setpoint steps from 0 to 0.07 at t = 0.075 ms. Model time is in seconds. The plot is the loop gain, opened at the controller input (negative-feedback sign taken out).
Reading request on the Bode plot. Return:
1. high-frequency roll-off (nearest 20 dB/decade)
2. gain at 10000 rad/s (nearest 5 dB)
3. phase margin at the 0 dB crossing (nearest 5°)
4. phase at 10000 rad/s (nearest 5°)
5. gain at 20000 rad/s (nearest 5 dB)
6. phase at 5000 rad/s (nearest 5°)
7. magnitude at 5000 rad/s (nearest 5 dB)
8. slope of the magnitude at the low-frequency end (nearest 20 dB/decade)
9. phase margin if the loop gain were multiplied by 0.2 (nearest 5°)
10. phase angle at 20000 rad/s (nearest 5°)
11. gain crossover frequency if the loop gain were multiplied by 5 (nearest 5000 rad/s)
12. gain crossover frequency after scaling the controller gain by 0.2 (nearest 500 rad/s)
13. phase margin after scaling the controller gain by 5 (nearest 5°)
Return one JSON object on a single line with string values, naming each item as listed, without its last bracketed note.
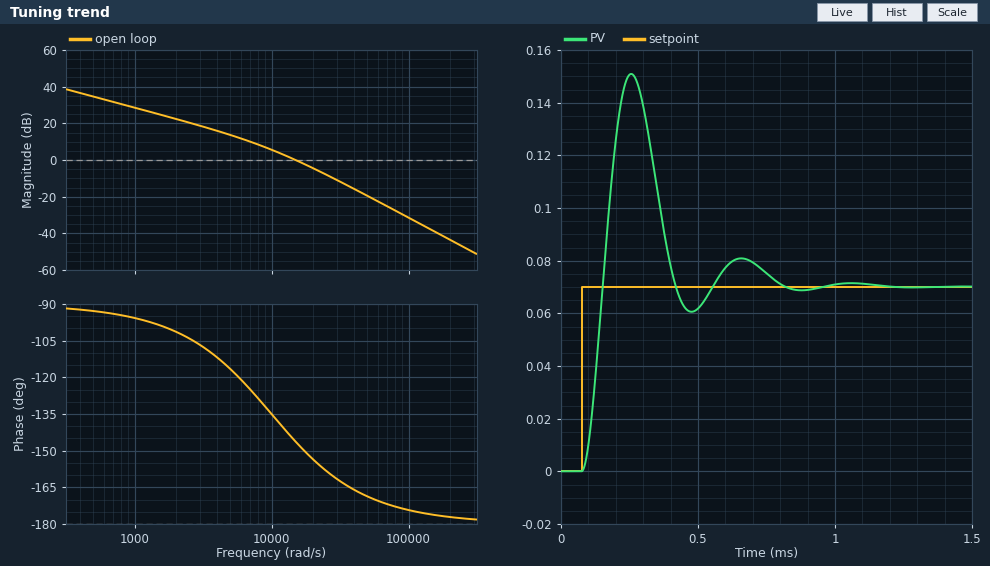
{"high-frequency roll-off": "-40 dB/decade", "gain at 10000 rad/s": "5 dB", "phase margin at the 0 dB crossing": "35°", "phase at 10000 rad/s": "-135°", "gain at 20000 rad/s": "-5 dB", "phase at 5000 rad/s": "-115°", "magnitude at 5000 rad/s": "15 dB", "slope of the magnitude at the low-frequency end": "-20 dB/decade", "phase margin if the loop gain were multiplied by 0.2": "65°", "phase angle at 20000 rad/s": "-155°", "gain crossover frequency if the loop gain were multiplied by 5": "35000 rad/s", "gain crossover frequency after scaling the controller gain by 0.2": "5000 rad/s", "phase margin after scaling the controller gain by 5": "15°"}
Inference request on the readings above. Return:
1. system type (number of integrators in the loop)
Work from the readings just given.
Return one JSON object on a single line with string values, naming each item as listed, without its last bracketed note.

{"system type": "1"}
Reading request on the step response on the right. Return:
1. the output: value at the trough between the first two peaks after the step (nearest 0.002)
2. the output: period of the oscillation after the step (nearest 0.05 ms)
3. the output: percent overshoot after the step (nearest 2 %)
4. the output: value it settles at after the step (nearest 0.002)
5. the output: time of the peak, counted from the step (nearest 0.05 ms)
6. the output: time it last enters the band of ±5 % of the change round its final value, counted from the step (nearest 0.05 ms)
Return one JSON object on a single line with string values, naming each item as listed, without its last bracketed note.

{"the output: value at the trough between the first two peaks after the step": "0.060", "the output: period of the oscillation after the step": "0.40 ms", "the output: percent overshoot after the step": "116 %", "the output: value it settles at after the step": "0.070", "the output: time of the peak, counted from the step": "0.20 ms", "the output: time it last enters the band of ±5 % of the change round its final value, counted from the step": "0.70 ms"}
